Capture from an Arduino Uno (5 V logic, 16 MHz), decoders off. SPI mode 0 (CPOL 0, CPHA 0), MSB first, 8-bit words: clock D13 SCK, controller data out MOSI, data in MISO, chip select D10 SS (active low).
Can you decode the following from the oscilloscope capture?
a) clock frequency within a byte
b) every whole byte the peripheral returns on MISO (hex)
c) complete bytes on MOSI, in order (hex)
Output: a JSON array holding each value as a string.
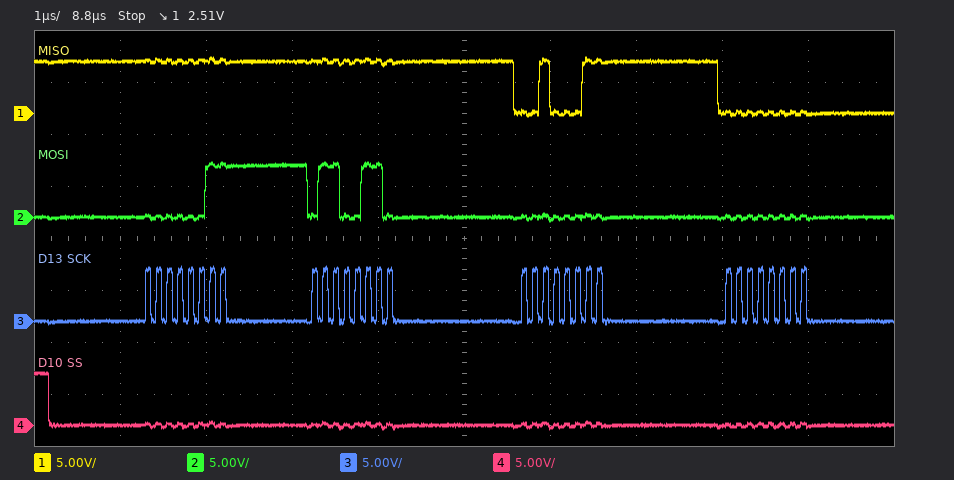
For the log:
["8 MHz", "FF FF 23 00", "03 66 00 00"]
